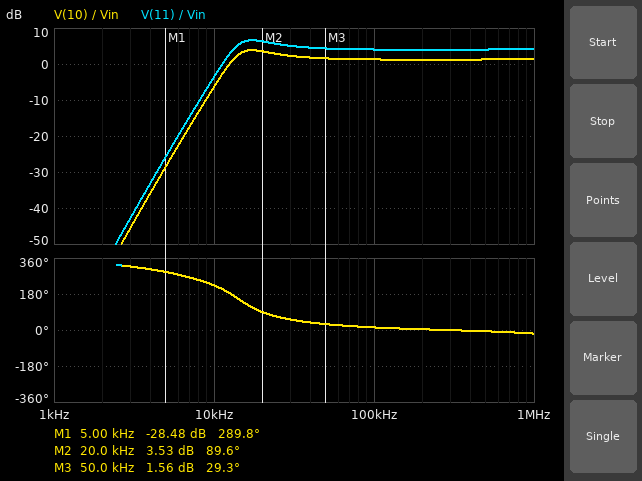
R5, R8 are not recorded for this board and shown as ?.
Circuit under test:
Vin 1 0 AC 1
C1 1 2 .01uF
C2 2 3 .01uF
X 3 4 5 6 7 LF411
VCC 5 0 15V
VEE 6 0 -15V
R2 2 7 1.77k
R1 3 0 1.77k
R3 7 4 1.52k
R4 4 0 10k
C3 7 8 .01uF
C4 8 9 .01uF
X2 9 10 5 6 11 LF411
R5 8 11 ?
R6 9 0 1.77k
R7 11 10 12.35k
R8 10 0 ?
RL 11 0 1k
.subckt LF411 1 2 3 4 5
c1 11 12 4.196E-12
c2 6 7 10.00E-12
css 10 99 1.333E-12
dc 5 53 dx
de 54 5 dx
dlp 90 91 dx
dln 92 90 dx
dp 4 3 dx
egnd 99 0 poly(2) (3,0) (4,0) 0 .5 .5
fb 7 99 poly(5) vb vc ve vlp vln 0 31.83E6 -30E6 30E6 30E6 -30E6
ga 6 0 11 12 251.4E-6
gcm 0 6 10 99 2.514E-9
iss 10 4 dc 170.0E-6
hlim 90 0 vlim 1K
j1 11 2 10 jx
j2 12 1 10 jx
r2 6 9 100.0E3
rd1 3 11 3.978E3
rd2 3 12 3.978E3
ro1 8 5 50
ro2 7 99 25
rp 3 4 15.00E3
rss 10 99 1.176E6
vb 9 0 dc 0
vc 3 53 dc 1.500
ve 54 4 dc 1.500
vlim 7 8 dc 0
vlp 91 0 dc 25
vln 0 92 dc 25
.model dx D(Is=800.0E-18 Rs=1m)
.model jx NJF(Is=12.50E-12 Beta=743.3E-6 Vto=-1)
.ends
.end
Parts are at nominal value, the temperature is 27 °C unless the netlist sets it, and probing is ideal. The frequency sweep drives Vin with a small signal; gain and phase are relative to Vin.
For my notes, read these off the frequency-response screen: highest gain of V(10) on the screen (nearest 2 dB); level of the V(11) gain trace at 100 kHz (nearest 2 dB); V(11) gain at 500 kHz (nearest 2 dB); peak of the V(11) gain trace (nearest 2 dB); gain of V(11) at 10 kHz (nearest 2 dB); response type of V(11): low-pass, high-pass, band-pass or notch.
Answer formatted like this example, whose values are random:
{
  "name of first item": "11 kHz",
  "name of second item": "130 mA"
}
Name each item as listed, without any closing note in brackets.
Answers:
{
  "highest gain of V(10) on the screen": "4 dB",
  "level of the V(11) gain trace at 100 kHz": "4 dB",
  "V(11) gain at 500 kHz": "4 dB",
  "peak of the V(11) gain trace": "6 dB",
  "gain of V(11) at 10 kHz": "-4 dB",
  "response type of V(11): low-pass, high-pass, band-pass or notch": "high-pass"
}
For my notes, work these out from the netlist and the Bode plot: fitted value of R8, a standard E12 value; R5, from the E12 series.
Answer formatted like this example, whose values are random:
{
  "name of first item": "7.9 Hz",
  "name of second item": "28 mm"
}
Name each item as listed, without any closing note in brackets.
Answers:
{
  "fitted value of R8, a standard E12 value": "33 kΩ",
  "R5, from the E12 series": "680 Ω"
}
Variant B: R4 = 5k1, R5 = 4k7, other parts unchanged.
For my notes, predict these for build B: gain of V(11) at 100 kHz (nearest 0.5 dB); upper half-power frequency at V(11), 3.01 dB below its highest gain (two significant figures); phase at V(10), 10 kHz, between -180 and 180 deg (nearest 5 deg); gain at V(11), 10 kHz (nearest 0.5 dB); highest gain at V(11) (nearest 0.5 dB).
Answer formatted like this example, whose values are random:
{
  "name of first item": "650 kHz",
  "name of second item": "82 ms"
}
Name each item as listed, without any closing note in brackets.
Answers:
{
  "gain of V(11) at 100 kHz": "5.0 dB",
  "upper half-power frequency at V(11), 3.01 dB below its highest gain": "5.4 MHz",
  "phase at V(10), 10 kHz, between -180 and 180 deg": "150 deg",
  "gain at V(11), 10 kHz": "-4.0 dB",
  "highest gain at V(11)": "8.5 dB"
}
